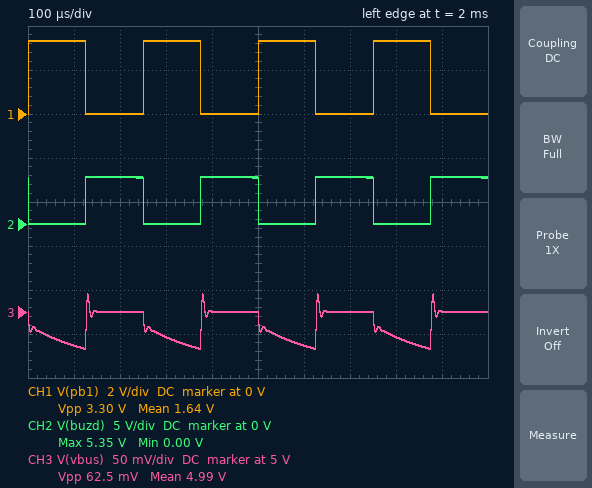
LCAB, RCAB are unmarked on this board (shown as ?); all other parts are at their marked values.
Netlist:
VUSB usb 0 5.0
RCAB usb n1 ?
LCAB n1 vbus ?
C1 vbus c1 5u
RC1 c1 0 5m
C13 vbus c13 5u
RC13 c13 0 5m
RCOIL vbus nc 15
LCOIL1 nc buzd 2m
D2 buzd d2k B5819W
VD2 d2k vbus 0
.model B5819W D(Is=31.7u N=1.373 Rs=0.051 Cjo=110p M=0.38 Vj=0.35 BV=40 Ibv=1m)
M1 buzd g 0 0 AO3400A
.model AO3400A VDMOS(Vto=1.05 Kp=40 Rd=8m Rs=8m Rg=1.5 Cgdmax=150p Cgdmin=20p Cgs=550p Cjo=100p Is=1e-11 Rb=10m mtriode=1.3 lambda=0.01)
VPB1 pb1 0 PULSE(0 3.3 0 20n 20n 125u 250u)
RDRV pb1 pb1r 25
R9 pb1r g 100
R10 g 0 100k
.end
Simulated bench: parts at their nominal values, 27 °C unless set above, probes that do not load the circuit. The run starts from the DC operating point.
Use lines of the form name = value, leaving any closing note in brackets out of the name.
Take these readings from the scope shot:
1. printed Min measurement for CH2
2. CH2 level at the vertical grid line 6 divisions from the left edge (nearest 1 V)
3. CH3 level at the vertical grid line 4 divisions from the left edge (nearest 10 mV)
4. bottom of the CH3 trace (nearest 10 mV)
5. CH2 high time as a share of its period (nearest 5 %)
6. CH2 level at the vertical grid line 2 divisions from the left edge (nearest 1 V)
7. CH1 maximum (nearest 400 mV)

printed Min measurement for CH2 = 0.00 V
CH2 level at the vertical grid line 6 divisions from the left edge = 0 V
CH3 level at the vertical grid line 4 divisions from the left edge = 5.00 V
bottom of the CH3 trace = 4.96 V
CH2 high time as a share of its period = 50 %
CH2 level at the vertical grid line 2 divisions from the left edge = 5 V
CH1 maximum = 3.2 V
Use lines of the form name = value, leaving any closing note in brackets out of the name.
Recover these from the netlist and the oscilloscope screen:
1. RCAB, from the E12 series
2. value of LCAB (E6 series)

RCAB, from the E12 series = 0.18 Ω
value of LCAB = 470 nH
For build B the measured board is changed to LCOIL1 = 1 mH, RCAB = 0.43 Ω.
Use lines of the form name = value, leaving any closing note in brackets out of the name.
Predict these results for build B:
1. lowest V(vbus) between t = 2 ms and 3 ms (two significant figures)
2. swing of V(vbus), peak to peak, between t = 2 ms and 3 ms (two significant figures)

lowest V(vbus) between t = 2 ms and 3 ms = 4.9 V
swing of V(vbus), peak to peak, between t = 2 ms and 3 ms = 120 mV
